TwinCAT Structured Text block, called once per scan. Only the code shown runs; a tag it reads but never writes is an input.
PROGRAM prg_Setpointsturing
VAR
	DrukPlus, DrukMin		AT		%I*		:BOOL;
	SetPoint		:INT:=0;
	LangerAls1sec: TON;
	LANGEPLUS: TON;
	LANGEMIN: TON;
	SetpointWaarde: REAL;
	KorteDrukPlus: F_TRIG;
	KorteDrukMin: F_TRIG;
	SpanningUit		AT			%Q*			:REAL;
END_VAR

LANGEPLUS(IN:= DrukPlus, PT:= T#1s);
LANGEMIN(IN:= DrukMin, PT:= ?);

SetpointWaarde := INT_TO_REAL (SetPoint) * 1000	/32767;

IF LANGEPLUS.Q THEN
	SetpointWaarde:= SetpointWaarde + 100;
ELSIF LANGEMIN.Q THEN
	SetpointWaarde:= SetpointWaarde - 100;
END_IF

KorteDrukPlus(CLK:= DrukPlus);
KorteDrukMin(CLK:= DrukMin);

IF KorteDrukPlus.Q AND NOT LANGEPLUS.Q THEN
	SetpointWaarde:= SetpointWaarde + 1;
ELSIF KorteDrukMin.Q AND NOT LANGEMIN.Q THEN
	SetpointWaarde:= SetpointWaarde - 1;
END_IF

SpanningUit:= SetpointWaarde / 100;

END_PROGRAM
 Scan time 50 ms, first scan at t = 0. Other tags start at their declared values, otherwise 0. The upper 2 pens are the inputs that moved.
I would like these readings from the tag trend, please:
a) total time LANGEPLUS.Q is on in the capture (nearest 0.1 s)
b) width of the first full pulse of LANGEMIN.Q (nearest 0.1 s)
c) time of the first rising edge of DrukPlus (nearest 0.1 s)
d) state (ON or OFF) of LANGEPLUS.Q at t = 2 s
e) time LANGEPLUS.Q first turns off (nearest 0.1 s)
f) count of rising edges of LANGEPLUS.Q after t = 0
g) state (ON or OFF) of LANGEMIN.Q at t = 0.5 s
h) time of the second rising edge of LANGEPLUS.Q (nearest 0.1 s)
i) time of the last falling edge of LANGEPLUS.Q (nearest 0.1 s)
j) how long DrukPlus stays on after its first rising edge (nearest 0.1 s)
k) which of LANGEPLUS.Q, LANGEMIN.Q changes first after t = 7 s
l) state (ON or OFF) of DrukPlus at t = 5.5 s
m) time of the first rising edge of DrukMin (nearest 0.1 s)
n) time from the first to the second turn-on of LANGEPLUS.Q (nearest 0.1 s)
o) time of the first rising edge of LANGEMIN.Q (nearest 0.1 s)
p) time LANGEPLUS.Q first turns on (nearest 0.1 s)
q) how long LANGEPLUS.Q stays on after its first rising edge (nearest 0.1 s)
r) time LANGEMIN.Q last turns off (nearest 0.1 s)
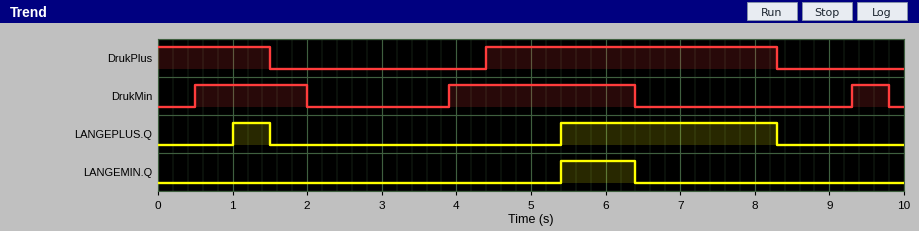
3.4 s
1.0 s
4.4 s
OFF
1.5 s
2
OFF
5.4 s
8.3 s
3.9 s
LANGEPLUS.Q
ON
0.5 s
4.4 s
5.4 s
1.0 s
0.5 s
6.4 s
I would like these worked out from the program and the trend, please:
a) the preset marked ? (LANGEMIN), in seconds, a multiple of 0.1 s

1.5 s
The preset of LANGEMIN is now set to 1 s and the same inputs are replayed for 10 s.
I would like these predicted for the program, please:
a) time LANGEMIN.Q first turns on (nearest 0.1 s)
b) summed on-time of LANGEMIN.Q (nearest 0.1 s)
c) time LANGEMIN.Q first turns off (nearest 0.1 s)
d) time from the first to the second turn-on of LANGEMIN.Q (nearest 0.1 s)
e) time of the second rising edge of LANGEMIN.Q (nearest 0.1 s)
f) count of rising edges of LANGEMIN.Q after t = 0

1.5 s
2.0 s
2.0 s
3.4 s
4.9 s
2
